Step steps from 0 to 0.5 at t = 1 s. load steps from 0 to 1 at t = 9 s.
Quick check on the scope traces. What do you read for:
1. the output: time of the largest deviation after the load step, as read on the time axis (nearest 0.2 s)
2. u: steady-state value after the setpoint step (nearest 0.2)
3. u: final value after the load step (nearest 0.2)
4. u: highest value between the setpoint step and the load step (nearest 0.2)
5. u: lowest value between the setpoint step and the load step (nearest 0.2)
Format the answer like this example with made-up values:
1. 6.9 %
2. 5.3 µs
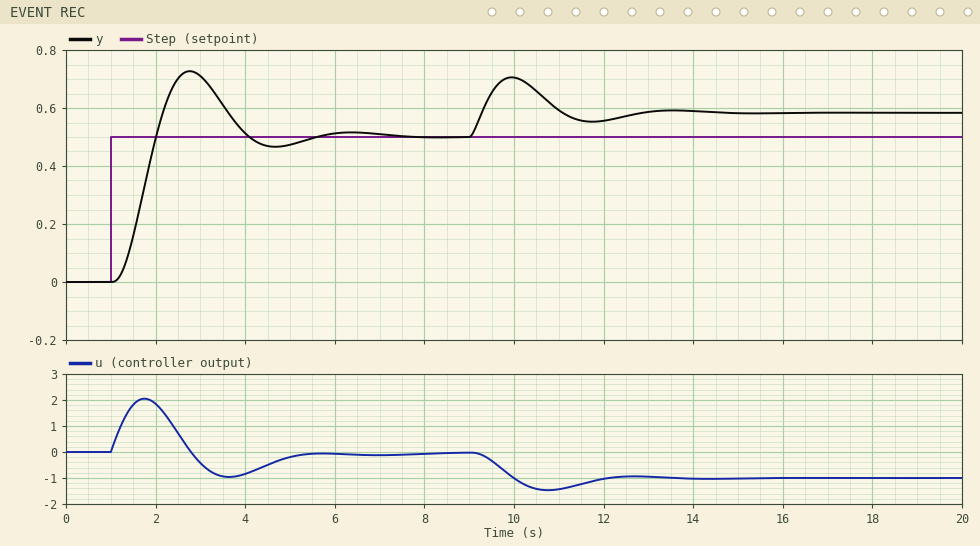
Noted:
1. 10.0 s
2. 0.0
3. -1.0
4. 2.0
5. -1.0
